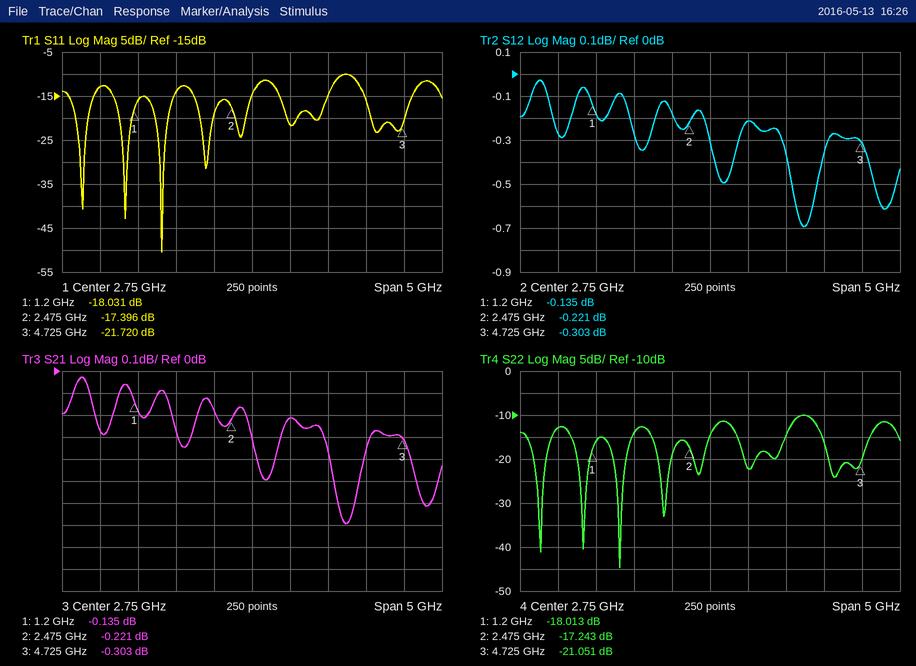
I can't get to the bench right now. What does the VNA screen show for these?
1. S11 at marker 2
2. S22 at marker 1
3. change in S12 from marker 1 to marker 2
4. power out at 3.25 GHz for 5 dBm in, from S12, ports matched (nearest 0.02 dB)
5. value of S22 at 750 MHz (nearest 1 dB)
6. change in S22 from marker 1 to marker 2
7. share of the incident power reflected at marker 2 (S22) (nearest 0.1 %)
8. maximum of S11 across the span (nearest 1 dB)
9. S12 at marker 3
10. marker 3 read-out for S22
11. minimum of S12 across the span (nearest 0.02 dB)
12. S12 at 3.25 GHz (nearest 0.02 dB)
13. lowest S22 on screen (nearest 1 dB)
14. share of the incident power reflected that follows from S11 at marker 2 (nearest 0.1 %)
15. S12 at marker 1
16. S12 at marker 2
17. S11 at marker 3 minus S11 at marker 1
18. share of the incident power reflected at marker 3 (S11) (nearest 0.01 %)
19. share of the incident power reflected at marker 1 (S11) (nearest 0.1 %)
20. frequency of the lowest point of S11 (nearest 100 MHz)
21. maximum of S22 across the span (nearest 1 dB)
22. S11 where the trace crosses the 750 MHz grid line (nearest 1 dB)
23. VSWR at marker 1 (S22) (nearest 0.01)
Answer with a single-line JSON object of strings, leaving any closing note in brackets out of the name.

{"S11 at marker 2": "-17.396 dB", "S22 at marker 1": "-18.013 dB", "change in S12 from marker 1 to marker 2": "-0.086 dB", "power out at 3.25 GHz for 5 dBm in, from S12, ports matched": "4.78 dBm", "value of S22 at 750 MHz": "-13 dB", "change in S22 from marker 1 to marker 2": "0.770 dB", "share of the incident power reflected at marker 2 (S22)": "1.9 %", "maximum of S11 across the span": "-10 dB", "S12 at marker 3": "-0.303 dB", "marker 3 read-out for S22": "-21.051 dB", "minimum of S12 across the span": "-0.70 dB", "S12 at 3.25 GHz": "-0.22 dB", "lowest S22 on screen": "-45 dB", "share of the incident power reflected that follows from S11 at marker 2": "1.8 %", "S12 at marker 1": "-0.135 dB", "S12 at marker 2": "-0.221 dB", "S11 at marker 3 minus S11 at marker 1": "-3.689 dB", "share of the incident power reflected at marker 3 (S11)": "0.67 %", "share of the incident power reflected at marker 1 (S11)": "1.6 %", "frequency of the lowest point of S11": "1.6 GHz", "maximum of S22 across the span": "-10 dB", "S11 where the trace crosses the 750 MHz grid line": "-13 dB", "VSWR at marker 1 (S22)": "1.29"}
